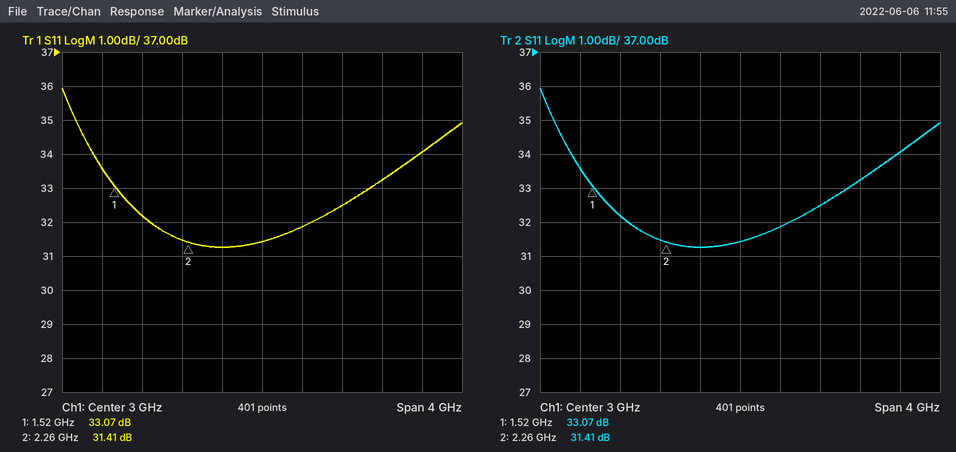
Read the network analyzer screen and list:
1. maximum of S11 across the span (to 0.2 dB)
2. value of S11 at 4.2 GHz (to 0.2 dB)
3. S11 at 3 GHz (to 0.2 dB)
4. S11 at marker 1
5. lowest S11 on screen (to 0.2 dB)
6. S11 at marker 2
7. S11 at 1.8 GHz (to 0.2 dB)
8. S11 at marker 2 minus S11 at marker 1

36.0 dB
33.2 dB
31.4 dB
33.07 dB
31.2 dB
31.41 dB
32.2 dB
-1.66 dB
